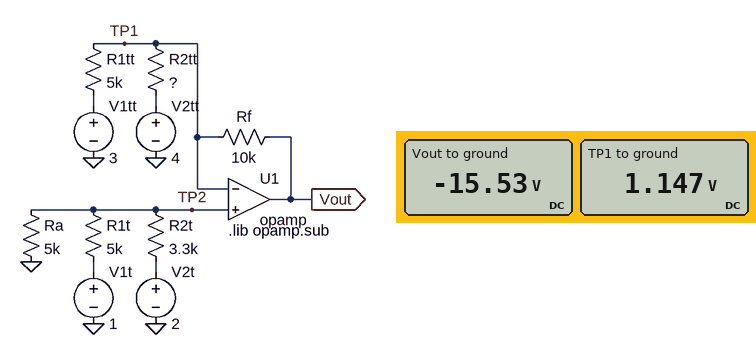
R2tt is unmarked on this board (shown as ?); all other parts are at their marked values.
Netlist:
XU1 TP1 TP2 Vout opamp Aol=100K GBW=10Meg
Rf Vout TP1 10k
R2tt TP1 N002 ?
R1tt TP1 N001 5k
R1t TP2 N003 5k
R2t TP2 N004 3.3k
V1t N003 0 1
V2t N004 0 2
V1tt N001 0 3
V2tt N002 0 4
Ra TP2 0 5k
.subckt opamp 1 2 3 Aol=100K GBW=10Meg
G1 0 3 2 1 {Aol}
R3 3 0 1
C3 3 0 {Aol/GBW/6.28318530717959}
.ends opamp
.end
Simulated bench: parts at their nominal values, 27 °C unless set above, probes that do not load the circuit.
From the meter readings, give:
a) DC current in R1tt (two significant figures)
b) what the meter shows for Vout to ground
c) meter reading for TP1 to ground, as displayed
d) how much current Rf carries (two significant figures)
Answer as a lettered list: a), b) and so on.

a) 370 µA
b) -15.53 V
c) 1.147 V
d) 1.7 mA
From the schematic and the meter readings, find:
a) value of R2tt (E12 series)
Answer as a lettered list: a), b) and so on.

a) 2.2 kΩ
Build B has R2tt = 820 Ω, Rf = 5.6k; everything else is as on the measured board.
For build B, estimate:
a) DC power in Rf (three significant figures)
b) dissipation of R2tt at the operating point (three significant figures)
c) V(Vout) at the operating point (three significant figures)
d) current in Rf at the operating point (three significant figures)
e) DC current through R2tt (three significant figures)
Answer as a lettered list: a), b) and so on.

a) 83.0 mW
b) 9.93 mW
c) -20.4 V
d) 3.85 mA
e) 3.48 mA
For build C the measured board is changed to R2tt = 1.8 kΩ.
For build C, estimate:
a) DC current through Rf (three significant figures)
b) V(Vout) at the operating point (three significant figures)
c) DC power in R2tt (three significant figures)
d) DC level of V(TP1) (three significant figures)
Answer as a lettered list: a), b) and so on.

a) 1.96 mA
b) -18.4 V
c) 4.52 mW
d) 1.15 V
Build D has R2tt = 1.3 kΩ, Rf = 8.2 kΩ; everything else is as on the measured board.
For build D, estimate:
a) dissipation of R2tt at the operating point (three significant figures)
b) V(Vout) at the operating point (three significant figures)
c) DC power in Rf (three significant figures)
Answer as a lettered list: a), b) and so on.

a) 6.26 mW
b) -19.9 V
c) 54.0 mW
